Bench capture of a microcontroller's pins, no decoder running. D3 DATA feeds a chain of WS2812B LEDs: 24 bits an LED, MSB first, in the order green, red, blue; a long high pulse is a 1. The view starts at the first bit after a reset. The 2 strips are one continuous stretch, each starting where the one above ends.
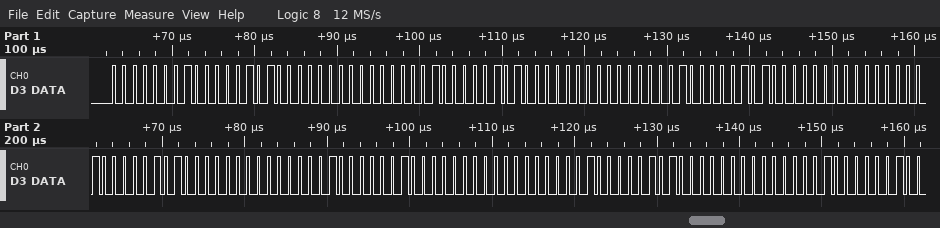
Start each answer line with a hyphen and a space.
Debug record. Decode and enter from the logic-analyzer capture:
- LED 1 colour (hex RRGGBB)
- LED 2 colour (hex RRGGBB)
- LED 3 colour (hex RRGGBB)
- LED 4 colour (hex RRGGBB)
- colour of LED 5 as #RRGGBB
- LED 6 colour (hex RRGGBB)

- #050100
- #050100
- #050100
- #050100
- #040200
- #050100
